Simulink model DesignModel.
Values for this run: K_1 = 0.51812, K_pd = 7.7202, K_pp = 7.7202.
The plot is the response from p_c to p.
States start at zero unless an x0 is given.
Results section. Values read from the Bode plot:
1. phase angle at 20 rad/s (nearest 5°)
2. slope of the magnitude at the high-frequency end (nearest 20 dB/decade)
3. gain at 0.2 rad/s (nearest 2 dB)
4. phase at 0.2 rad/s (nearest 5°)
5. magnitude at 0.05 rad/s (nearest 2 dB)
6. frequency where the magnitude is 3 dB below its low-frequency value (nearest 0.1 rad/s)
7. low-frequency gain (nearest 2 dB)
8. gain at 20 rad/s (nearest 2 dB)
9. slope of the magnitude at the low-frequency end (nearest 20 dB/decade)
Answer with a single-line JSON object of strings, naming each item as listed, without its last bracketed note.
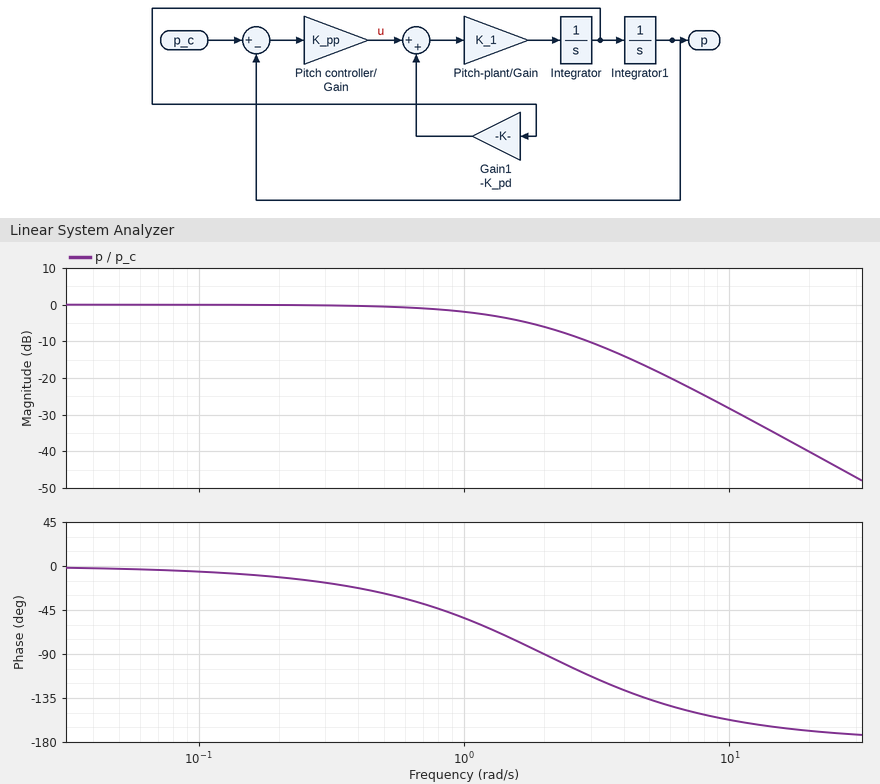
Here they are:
{"phase angle at 20 rad/s": "-170°", "slope of the magnitude at the high-frequency end": "-40 dB/decade", "gain at 0.2 rad/s": "0 dB", "phase at 0.2 rad/s": "-10°", "magnitude at 0.05 rad/s": "0 dB", "frequency where the magnitude is 3 dB below its low-frequency value": "1.3 rad/s", "low-frequency gain": "0 dB", "gain at 20 rad/s": "-40 dB", "slope of the magnitude at the low-frequency end": "0 dB/decade"}
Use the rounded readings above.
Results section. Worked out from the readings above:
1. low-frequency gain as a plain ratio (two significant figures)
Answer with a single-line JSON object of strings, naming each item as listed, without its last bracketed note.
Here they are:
{"low-frequency gain as a plain ratio": "1.0"}
